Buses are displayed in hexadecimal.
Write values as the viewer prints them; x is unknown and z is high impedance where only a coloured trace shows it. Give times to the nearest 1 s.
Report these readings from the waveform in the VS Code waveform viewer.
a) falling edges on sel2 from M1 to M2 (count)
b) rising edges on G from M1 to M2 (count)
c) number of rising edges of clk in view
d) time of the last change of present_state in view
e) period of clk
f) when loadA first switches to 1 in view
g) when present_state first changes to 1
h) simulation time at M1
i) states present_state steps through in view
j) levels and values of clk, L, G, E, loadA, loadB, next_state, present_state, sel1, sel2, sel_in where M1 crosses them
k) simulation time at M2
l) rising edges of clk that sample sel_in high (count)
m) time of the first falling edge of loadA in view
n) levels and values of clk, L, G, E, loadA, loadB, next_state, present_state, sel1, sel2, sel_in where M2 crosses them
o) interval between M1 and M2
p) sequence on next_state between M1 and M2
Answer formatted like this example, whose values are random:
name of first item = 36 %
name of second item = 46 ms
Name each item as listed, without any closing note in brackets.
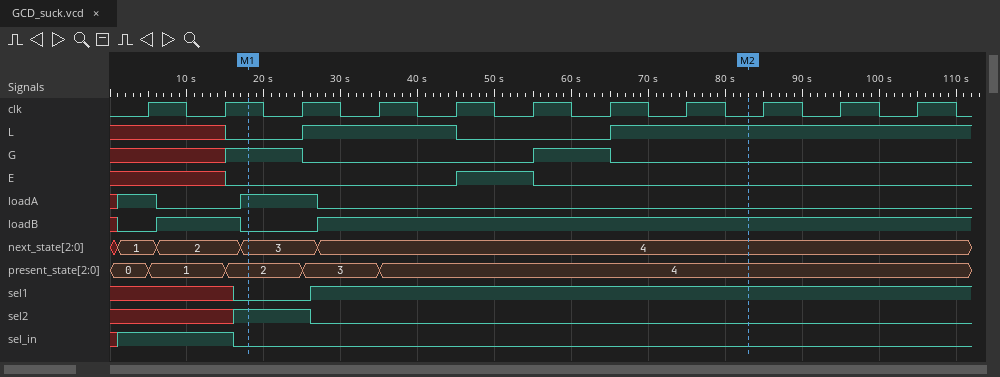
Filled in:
falling edges on sel2 from M1 to M2 = 1
rising edges on G from M1 to M2 = 1
number of rising edges of clk in view = 11
time of the last change of present_state in view = 35 s
period of clk = 10 s
when loadA first switches to 1 in view = 1 s
when present_state first changes to 1 = 5 s
simulation time at M1 = 18 s
states present_state steps through in view = 0, 1, 2, 3, 4
levels and values of clk, L, G, E, loadA, loadB, next_state, present_state, sel1, sel2, sel_in where M1 crosses them = clk=1, L=0, G=1, E=0, loadA=1, loadB=0, next_state=3, present_state=2, sel1=0, sel2=1, sel_in=0
simulation time at M2 = 83 s
rising edges of clk that sample sel_in high = 2
time of the first falling edge of loadA in view = 6 s
levels and values of clk, L, G, E, loadA, loadB, next_state, present_state, sel1, sel2, sel_in where M2 crosses them = clk=0, L=1, G=0, E=0, loadA=0, loadB=1, next_state=4, present_state=4, sel1=1, sel2=0, sel_in=0
interval between M1 and M2 = 65 s
sequence on next_state between M1 and M2 = 3, 4
